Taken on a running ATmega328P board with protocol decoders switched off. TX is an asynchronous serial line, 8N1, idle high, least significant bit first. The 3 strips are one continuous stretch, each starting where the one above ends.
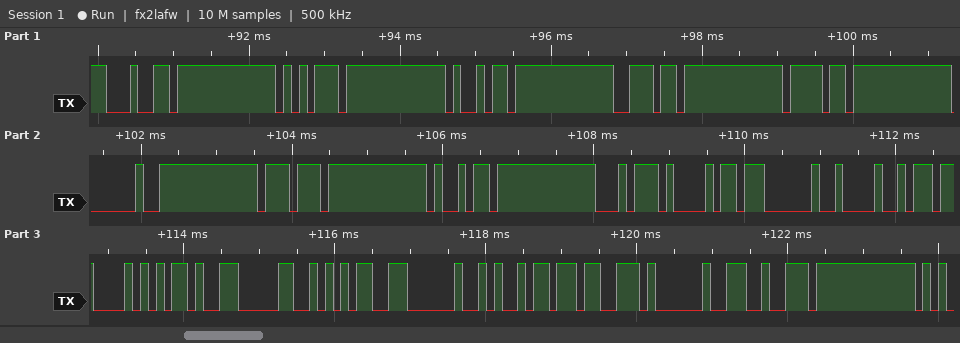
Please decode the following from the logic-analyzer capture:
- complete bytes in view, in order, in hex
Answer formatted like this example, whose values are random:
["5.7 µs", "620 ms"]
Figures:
["0x64 0x75 0x69 0x6E 0x6F 0x20 0x77 0x69 0x74 0x68 0x20 0x48 0x43 0x2D 0x30 0x35 0x20 0x69 0x73 0x20 0x72"]
